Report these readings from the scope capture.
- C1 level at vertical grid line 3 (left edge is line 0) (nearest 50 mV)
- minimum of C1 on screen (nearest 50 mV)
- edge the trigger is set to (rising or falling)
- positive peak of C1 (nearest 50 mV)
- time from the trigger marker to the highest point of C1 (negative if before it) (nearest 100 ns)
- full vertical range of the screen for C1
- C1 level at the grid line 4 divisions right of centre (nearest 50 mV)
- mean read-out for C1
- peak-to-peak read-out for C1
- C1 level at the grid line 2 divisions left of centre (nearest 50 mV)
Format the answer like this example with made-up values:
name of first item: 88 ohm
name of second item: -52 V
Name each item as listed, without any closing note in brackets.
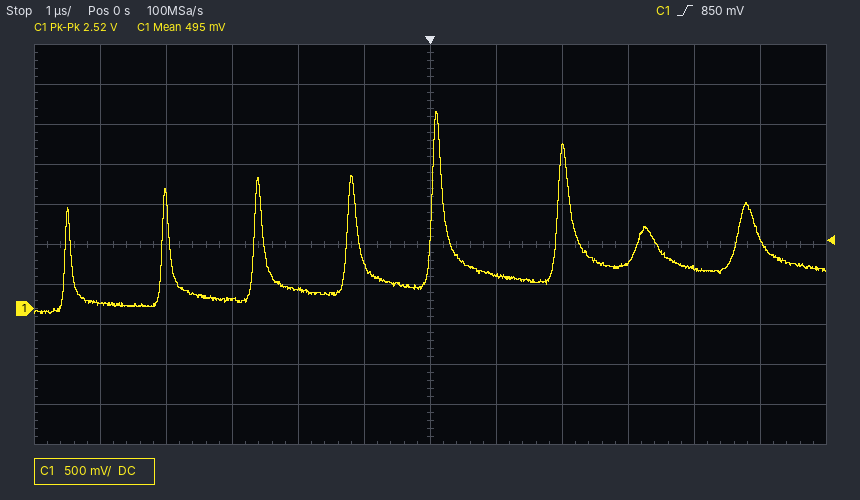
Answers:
C1 level at vertical grid line 3 (left edge is line 0): 100 mV
minimum of C1 on screen: -50 mV
edge the trigger is set to: rising
positive peak of C1: 2.45 V
time from the trigger marker to the highest point of C1 (negative if before it): +100 ns
full vertical range of the screen for C1: 5 V
C1 level at the grid line 4 divisions right of centre: 500 mV
mean read-out for C1: 495 mV
peak-to-peak read-out for C1: 2.52 V
C1 level at the grid line 2 divisions left of centre: 250 mV
